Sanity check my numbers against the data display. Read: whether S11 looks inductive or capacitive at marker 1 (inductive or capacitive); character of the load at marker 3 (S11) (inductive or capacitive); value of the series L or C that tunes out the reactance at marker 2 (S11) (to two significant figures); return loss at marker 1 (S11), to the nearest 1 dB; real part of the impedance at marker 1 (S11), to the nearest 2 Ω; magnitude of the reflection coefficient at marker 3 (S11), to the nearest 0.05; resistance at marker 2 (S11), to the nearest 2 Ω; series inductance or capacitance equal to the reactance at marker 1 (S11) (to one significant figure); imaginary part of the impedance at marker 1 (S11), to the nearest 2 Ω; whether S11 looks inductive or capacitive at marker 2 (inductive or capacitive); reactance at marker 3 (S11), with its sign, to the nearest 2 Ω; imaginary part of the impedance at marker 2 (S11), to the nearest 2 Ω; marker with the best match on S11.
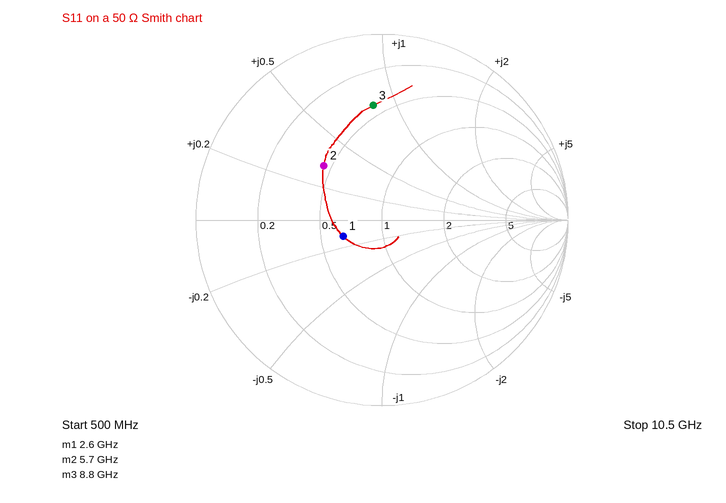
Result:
capacitive
inductive
1.7 pF
13 dB
32 Ω
0.60
22 Ω
10 pF
-6 Ω
inductive
+42 Ω
+16 Ω
marker 1
